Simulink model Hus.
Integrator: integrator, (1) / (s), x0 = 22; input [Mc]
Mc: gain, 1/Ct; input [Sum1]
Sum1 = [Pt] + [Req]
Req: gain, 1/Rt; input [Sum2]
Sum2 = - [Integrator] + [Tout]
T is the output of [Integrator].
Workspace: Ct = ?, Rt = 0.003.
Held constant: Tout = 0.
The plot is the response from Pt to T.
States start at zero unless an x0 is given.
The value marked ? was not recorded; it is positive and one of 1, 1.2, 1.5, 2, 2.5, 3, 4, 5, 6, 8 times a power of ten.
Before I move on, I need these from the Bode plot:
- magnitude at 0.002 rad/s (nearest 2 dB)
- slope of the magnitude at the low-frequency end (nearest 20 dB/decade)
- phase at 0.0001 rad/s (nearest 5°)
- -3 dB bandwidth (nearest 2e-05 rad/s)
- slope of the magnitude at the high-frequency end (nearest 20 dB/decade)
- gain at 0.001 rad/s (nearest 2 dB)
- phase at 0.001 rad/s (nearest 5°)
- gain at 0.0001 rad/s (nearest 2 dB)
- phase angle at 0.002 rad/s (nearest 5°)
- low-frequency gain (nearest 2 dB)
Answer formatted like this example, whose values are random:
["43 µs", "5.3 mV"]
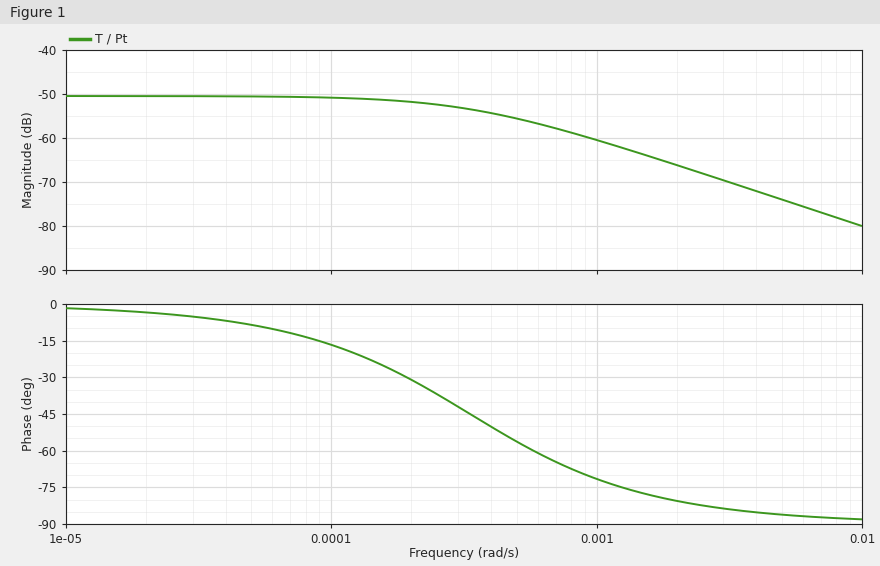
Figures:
["-66 dB", "0 dB/decade", "-15°", "0.00034 rad/s", "-20 dB/decade", "-60 dB", "-70°", "-50 dB", "-80°", "-50 dB"]
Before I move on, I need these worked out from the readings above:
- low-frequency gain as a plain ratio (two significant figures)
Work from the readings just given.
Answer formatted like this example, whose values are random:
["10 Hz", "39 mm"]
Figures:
["0.0032"]
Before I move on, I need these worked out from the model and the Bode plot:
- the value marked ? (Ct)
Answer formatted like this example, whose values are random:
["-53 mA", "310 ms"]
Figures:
["1e+06"]
